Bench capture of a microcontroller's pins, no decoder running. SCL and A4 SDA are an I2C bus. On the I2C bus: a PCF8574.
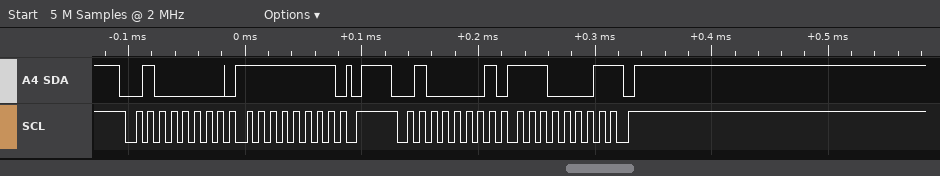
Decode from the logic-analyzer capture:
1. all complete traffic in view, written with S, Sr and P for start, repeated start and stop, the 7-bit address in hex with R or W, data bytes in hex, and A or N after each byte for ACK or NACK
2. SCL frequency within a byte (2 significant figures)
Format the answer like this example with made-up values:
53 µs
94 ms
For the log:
S 20W A FF A P S 20R A E1 N P
100 kHz
